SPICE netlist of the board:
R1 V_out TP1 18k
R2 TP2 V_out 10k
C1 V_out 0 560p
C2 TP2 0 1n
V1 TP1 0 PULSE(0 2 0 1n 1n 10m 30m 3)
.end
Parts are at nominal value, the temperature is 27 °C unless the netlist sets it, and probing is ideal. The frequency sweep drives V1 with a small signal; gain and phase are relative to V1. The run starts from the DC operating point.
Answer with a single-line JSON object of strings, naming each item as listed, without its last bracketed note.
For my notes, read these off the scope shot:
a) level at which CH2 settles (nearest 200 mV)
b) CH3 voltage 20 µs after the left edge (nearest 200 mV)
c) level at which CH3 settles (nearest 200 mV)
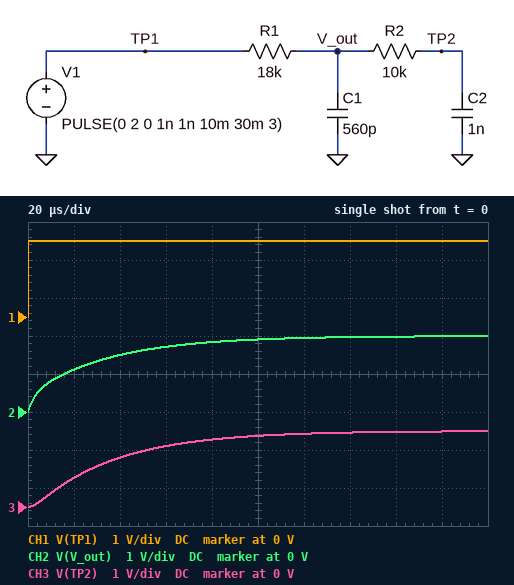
{"level at which CH2 settles": "2.0 V", "CH3 voltage 20 µs after the left edge": "800 mV", "level at which CH3 settles": "2.0 V"}
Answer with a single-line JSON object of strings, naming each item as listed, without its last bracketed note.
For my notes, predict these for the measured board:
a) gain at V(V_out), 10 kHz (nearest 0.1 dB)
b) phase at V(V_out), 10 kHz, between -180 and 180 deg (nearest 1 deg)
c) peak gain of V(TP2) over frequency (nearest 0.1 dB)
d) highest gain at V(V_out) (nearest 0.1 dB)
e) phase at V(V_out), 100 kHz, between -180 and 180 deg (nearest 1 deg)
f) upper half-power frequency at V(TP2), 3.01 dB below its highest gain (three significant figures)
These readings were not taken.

{"gain at V(V_out), 10 kHz": "-6.4 dB", "phase at V(V_out), 10 kHz, between -180 and 180 deg": "-44 deg", "peak gain of V(TP2) over frequency": "0 dB", "highest gain at V(V_out)": "0 dB", "phase at V(V_out), 100 kHz, between -180 and 180 deg": "-67 deg", "upper half-power frequency at V(TP2), 3.01 dB below its highest gain": "4.49 kHz"}
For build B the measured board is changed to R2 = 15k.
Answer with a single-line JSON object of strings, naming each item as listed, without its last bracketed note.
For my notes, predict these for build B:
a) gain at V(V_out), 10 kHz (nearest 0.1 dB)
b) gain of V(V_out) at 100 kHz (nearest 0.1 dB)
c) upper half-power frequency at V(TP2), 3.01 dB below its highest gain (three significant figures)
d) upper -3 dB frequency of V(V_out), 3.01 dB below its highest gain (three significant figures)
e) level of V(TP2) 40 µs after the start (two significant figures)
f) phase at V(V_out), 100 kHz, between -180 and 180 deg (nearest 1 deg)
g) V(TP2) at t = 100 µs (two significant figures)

{"gain at V(V_out), 10 kHz": "-6.0 dB", "gain of V(V_out) at 100 kHz": "-16.7 dB", "upper half-power frequency at V(TP2), 3.01 dB below its highest gain": "4.02 kHz", "upper -3 dB frequency of V(V_out), 3.01 dB below its highest gain": "4.75 kHz", "level of V(TP2) 40 µs after the start": "1.2 V", "phase at V(V_out), 100 kHz, between -180 and 180 deg": "-71 deg", "V(TP2) at t = 100 µs": "1.8 V"}
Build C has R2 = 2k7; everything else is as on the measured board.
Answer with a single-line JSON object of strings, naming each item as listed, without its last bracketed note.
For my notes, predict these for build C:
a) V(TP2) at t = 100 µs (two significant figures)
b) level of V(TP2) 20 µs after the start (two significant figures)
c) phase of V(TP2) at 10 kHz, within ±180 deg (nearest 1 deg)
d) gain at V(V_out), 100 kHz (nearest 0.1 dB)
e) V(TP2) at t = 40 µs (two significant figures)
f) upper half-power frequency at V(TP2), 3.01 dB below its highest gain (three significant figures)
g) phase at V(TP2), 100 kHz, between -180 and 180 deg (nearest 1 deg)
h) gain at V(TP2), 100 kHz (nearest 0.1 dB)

{"V(TP2) at t = 100 µs": "1.9 V", "level of V(TP2) 20 µs after the start": "940 mV", "phase of V(TP2) at 10 kHz, within ±180 deg": "-65 deg", "gain at V(V_out), 100 kHz": "-20.8 dB", "V(TP2) at t = 40 µs": "1.5 V", "upper half-power frequency at V(TP2), 3.01 dB below its highest gain": "5.32 kHz", "phase at V(TP2), 100 kHz, between -180 and 180 deg": "-117 deg", "gain at V(TP2), 100 kHz": "-26.7 dB"}
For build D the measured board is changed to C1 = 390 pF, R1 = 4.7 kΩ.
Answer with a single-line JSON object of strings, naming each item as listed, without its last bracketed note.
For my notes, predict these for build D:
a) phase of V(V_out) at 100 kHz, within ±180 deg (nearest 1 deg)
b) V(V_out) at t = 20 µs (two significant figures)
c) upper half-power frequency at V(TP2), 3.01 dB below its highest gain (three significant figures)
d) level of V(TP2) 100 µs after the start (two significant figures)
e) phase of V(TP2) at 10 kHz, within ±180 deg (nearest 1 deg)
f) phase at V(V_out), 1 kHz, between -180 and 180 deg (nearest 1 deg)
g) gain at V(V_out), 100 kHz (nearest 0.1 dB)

{"phase of V(V_out) at 100 kHz, within ±180 deg": "-40 deg", "V(V_out) at t = 20 µs": "1.8 V", "upper half-power frequency at V(TP2), 3.01 dB below its highest gain": "10.3 kHz", "level of V(TP2) 100 µs after the start": "2.0 V", "phase of V(TP2) at 10 kHz, within ±180 deg": "-48 deg", "phase at V(V_out), 1 kHz, between -180 and 180 deg": "-2 deg", "gain at V(V_out), 100 kHz": "-5.6 dB"}
